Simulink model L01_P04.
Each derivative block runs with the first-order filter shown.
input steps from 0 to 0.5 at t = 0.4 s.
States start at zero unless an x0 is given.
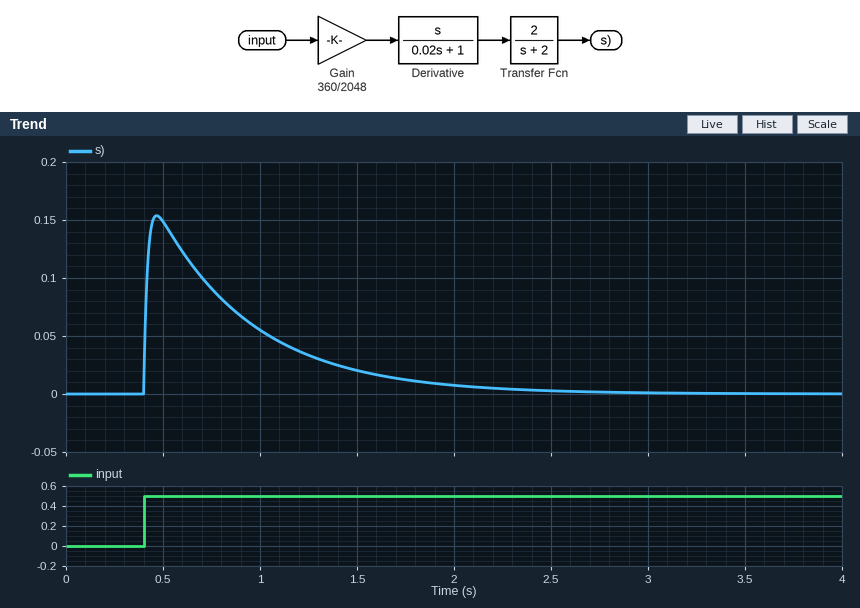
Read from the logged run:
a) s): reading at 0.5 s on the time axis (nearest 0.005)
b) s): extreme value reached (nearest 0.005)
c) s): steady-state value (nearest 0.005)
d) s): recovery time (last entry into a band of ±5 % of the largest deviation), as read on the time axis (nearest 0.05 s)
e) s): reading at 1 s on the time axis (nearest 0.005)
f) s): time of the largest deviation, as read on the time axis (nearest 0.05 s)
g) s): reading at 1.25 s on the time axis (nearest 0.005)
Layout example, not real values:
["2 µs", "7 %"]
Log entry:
["0.150", "0.155", "0.000", "2.00 s", "0.055", "0.45 s", "0.035"]
